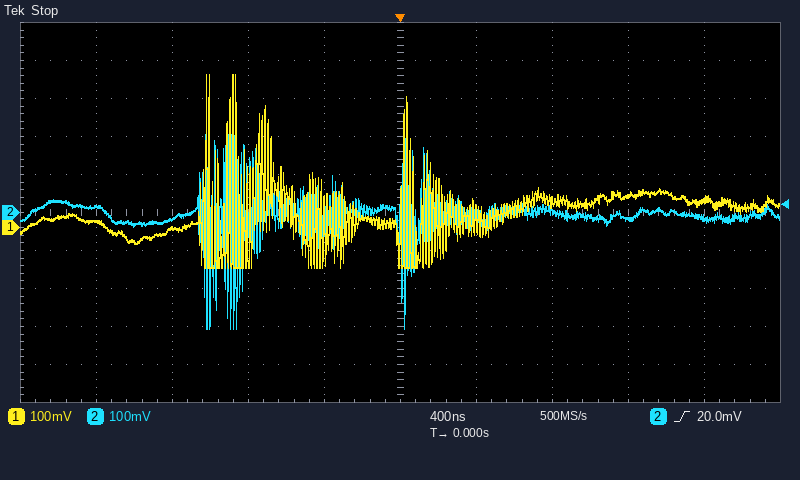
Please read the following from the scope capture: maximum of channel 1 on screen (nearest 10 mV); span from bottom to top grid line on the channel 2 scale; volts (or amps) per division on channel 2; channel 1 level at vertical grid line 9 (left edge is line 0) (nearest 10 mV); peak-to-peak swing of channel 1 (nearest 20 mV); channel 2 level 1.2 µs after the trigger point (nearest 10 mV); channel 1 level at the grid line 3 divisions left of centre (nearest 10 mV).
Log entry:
400 mV
1 V
100 mV
70 mV
500 mV
-20 mV
0 mV
